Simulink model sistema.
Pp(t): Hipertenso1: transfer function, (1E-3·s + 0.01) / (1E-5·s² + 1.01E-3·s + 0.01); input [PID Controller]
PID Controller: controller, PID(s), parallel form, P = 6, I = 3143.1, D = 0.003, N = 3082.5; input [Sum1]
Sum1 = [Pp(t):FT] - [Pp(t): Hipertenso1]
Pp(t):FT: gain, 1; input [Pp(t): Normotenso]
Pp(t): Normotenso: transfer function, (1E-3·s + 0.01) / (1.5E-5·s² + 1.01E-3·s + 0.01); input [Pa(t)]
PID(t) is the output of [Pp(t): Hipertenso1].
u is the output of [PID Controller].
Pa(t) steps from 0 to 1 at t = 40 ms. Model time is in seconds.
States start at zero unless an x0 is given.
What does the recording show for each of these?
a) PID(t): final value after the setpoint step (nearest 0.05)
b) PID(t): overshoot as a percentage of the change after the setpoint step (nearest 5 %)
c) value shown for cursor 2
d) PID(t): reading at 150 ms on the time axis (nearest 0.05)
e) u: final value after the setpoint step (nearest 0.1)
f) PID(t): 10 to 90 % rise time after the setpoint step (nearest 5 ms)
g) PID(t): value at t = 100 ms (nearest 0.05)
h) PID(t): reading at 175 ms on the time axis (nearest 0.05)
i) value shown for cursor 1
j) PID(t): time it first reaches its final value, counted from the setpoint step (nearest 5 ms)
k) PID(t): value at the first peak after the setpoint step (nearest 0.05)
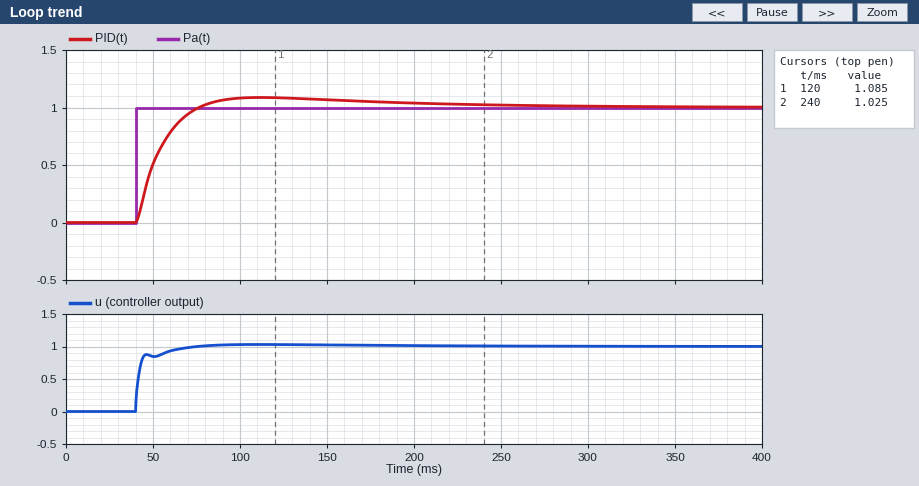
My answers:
1.00
10 %
1.025
1.05
1.0
25 ms
1.10
1.05
1.085
35 ms
1.10
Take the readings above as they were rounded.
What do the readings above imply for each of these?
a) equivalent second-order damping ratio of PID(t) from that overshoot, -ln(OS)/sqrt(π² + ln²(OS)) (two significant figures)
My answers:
0.59
